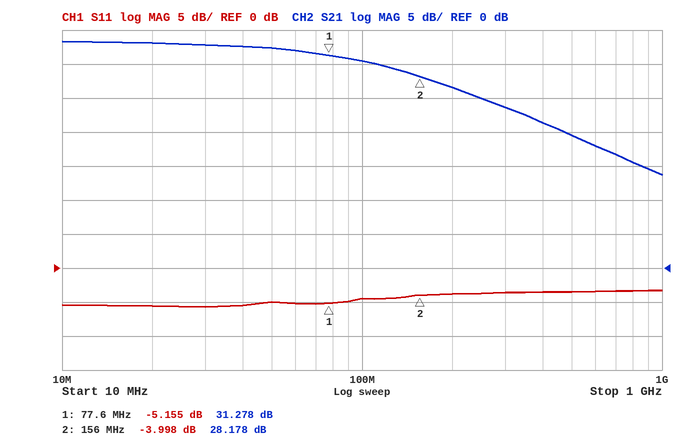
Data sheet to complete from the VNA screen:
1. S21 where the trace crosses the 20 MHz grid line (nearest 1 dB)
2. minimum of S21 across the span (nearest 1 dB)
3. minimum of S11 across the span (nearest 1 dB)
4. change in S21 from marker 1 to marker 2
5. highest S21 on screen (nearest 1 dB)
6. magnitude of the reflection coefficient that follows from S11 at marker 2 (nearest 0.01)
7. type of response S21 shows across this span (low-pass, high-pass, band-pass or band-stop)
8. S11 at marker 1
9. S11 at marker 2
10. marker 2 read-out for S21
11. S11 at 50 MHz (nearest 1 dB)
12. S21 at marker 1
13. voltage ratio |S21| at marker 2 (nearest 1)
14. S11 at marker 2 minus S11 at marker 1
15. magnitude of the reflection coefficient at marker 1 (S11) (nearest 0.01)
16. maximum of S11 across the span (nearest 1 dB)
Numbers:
33 dB
14 dB
-6 dB
-3.100 dB
33 dB
0.63
low-pass
-5.155 dB
-3.998 dB
28.178 dB
-5 dB
31.278 dB
26
1.157 dB
0.55
-3 dB
